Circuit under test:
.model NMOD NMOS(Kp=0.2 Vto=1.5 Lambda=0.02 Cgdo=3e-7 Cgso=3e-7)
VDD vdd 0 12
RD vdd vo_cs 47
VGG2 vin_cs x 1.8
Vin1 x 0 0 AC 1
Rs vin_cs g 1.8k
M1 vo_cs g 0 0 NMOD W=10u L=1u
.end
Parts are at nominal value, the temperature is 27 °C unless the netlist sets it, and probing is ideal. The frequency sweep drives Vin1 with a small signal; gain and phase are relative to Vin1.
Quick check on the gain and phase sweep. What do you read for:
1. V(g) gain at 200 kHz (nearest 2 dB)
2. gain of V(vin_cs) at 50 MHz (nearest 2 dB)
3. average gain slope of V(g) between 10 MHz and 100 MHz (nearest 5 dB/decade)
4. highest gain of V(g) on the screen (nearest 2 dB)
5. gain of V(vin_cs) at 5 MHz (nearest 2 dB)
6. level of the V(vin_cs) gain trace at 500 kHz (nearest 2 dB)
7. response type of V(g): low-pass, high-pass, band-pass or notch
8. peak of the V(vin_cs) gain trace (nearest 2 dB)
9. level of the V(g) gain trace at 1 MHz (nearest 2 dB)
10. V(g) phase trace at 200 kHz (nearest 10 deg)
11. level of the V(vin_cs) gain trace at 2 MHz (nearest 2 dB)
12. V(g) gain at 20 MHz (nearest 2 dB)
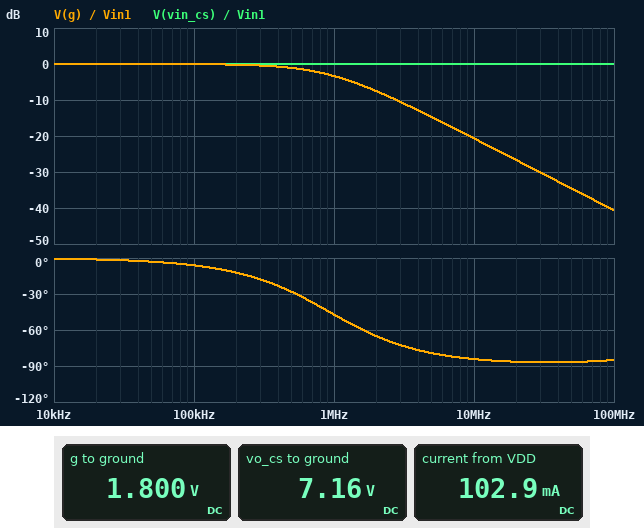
0 dB
0 dB
-20 dB/decade
0 dB
0 dB
0 dB
low-pass
0 dB
-4 dB
-10 deg
0 dB
-26 dB
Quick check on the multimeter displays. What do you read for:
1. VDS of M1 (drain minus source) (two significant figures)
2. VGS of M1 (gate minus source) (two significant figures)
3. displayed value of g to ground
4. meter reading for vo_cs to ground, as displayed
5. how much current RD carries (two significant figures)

7.2 V
1.8 V
1.800 V
7.16 V
100 mA
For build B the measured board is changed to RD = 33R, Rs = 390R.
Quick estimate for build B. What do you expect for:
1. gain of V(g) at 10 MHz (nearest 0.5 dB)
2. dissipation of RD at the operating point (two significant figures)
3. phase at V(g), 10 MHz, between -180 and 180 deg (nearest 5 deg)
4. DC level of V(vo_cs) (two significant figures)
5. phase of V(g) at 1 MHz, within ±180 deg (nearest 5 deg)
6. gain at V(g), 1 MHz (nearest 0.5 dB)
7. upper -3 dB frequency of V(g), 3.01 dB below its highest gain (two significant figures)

-6.0 dB
370 mW
-60 deg
8.5 V
-10 deg
0 dB
5.7 MHz
